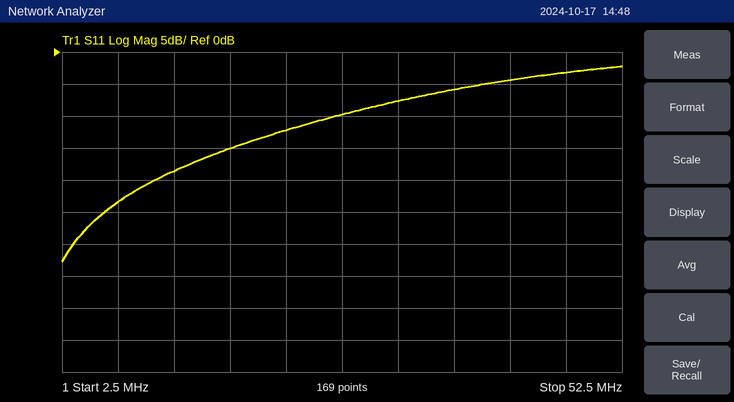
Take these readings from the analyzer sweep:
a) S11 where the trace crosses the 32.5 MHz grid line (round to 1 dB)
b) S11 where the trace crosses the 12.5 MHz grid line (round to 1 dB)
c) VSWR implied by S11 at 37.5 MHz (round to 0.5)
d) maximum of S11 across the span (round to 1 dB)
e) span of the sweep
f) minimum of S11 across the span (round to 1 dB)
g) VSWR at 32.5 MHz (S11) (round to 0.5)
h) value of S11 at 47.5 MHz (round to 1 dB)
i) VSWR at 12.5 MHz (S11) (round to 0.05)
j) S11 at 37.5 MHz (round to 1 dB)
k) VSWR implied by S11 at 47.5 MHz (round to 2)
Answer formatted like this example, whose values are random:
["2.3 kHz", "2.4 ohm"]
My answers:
["-8 dB", "-19 dB", "3.0", "-2 dB", "50 MHz", "-33 dB", "2.5", "-3 dB", "1.25", "-6 dB", "6"]
